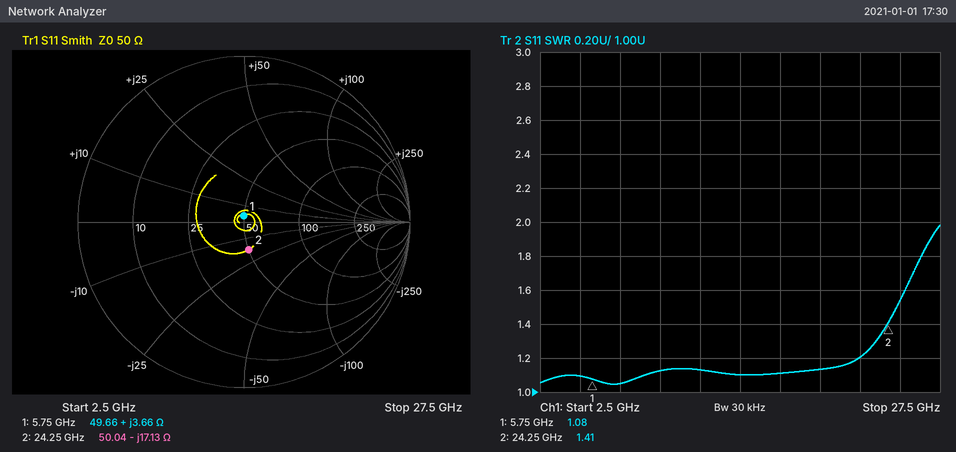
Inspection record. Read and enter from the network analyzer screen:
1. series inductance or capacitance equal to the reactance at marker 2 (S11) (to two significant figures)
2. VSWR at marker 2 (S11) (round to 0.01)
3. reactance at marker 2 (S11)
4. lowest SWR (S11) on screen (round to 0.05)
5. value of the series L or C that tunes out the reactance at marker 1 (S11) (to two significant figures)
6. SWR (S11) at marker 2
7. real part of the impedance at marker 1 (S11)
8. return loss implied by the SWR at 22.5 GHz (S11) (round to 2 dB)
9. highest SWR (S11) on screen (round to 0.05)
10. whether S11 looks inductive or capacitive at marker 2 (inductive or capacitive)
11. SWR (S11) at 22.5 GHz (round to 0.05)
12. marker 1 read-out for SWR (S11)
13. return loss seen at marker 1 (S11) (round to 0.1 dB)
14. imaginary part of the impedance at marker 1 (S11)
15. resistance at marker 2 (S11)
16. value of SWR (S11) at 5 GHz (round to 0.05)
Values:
380 fF
1.41
-17.13 Ω
1.05
7.6 pF
1.41
49.66 Ω
20 dB
2.00
capacitive
1.20
1.08
28.7 dB
+3.66 Ω
50.04 Ω
1.10
